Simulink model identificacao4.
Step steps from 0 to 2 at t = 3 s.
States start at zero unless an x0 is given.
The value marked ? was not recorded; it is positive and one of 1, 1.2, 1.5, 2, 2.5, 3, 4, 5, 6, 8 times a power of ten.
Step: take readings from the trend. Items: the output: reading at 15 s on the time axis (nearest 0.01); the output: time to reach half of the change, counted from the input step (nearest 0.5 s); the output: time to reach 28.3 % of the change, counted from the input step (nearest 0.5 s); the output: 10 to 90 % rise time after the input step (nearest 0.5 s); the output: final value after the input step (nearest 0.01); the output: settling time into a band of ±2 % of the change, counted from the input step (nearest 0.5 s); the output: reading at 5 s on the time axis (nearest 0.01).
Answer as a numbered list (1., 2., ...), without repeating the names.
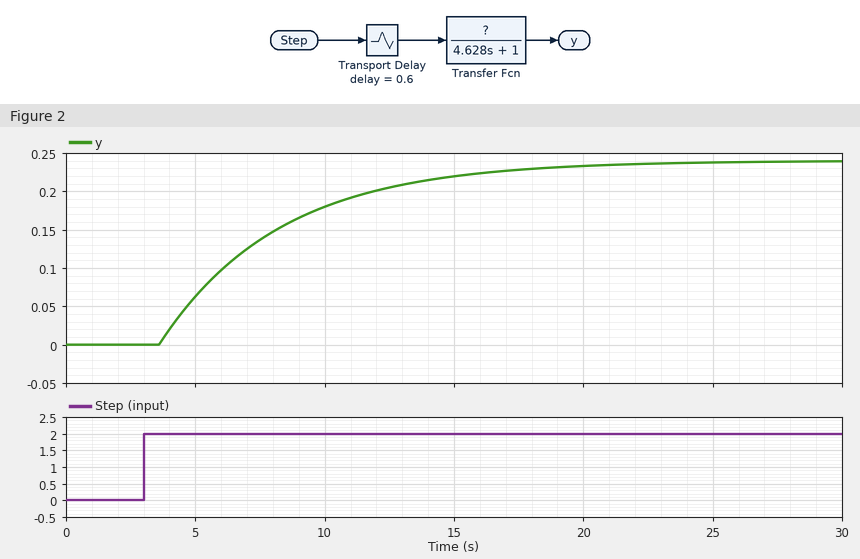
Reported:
1. 0.22
2. 4.0 s
3. 2.0 s
4. 10.0 s
5. 0.24
6. 18.5 s
7. 0.06
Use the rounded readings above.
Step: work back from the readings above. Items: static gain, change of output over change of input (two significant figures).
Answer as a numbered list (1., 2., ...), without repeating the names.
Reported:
1. 0.12
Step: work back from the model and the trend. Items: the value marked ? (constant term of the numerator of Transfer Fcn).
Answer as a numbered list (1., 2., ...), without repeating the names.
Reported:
1. 0.12
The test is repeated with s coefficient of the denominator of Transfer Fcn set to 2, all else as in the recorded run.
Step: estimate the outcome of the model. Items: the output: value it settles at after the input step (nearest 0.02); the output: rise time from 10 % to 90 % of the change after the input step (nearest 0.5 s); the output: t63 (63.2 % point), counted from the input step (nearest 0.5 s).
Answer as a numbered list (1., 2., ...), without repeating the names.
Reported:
1. 0.24
2. 4.5 s
3. 2.5 s
